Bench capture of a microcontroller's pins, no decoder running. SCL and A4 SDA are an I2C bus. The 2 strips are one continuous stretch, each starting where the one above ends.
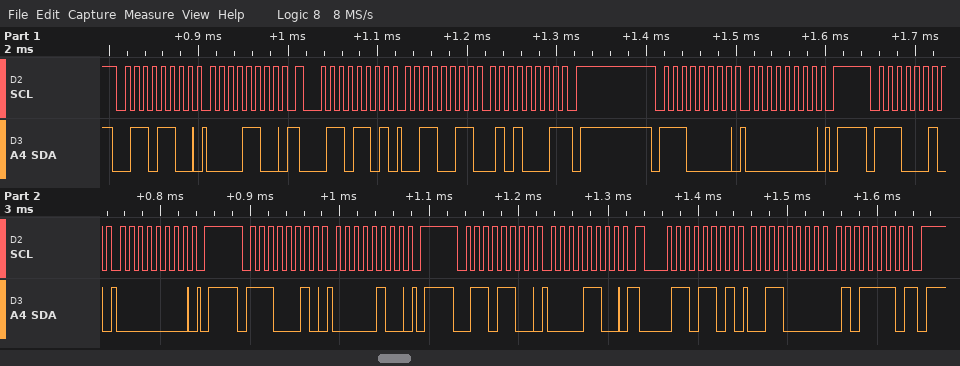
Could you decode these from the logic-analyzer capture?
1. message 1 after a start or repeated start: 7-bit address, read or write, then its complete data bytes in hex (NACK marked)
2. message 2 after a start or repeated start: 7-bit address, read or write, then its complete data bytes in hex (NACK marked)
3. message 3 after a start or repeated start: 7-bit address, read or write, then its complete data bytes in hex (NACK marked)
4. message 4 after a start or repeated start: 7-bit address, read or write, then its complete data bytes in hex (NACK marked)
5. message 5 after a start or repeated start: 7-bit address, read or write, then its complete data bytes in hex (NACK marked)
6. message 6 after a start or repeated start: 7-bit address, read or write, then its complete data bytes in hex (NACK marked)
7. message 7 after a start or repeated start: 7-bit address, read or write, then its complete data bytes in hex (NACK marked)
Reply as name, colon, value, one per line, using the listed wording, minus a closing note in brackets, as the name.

message 1 after a start or repeated start: 7-bit address, read or write, then its complete data bytes in hex: 0x36 write: 0C
message 2 after a start or repeated start: 7-bit address, read or write, then its complete data bytes in hex: 0x36 read: 33 51 NACK
message 3 after a start or repeated start: 7-bit address, read or write, then its complete data bytes in hex: 0x70 write: 00
message 4 after a start or repeated start: 7-bit address, read or write, then its complete data bytes in hex: 0x71 write: 00
message 5 after a start or repeated start: 7-bit address, read or write, then its complete data bytes in hex: 0x71 write: 04
message 6 after a start or repeated start: 7-bit address, read or write, then its complete data bytes in hex: 0x36 write: 0C
message 7 after a start or repeated start: 7-bit address, read or write, then its complete data bytes in hex: 0x36 read: 30 5E NACK
